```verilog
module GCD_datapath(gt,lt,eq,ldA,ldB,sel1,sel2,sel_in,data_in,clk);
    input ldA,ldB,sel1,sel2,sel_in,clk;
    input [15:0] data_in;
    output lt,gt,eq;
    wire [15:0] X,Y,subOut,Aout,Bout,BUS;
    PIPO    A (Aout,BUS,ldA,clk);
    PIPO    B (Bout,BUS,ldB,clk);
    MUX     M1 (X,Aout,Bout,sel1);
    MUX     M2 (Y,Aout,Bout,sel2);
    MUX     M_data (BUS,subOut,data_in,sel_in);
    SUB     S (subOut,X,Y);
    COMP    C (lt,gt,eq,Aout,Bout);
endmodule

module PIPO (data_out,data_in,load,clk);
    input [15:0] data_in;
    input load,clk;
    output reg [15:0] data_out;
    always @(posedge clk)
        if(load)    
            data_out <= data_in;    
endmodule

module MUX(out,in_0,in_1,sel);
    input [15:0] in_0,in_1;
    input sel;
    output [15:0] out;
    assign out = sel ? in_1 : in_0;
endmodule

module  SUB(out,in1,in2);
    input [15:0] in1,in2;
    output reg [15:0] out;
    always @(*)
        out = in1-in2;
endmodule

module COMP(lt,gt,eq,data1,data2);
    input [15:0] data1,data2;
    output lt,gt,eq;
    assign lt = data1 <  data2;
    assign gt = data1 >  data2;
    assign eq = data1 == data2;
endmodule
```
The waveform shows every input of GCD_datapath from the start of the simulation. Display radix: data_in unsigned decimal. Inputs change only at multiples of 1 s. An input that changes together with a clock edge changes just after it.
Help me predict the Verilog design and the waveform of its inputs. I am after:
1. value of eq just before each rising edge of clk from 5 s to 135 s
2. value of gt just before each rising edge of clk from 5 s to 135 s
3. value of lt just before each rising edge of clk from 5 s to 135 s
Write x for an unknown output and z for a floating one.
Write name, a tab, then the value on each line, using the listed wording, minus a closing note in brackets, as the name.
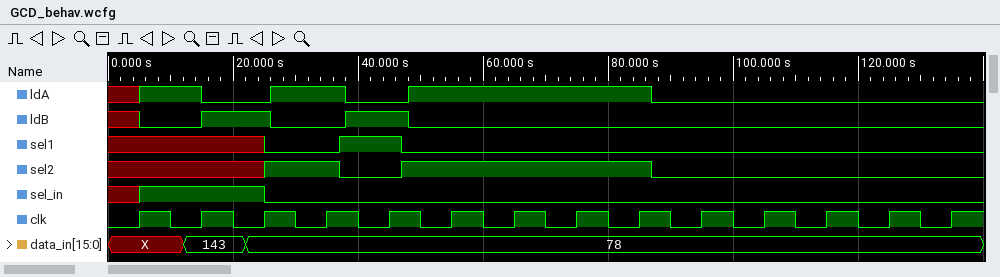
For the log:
value of eq just before each rising edge of clk from 5 s to 135 s	x x x 0 0 0 0 0 0 1 1 1 1 1
value of gt just before each rising edge of clk from 5 s to 135 s	x x x 1 0 1 1 1 1 0 0 0 0 0
value of lt just before each rising edge of clk from 5 s to 135 s	x x x 0 1 0 0 0 0 0 0 0 0 0
